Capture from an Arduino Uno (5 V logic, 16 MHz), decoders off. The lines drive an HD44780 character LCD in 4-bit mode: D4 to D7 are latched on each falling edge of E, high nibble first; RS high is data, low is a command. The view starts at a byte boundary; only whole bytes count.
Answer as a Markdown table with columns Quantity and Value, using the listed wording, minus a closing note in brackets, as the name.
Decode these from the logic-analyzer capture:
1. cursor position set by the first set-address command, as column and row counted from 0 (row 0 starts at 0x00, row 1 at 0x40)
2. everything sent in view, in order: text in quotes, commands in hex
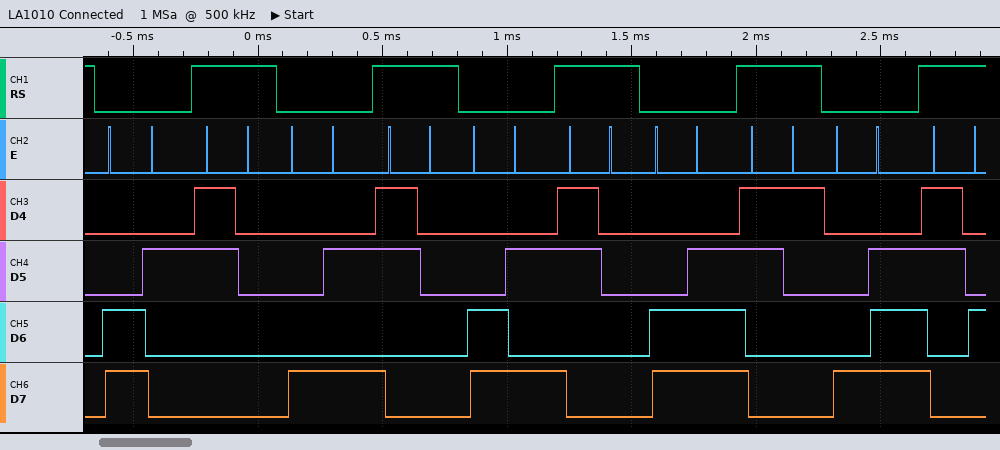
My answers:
| Quantity | Value |
|---|---|
| cursor position set by the first set-address command, as column and row counted from 0 | column 2, row 1 |
| everything sent in view, in order: text in quotes, commands in hex | 0xC2 "0" 0x8A "0" 0xCA "0" 0xCE "1" 0x8E "4" |
